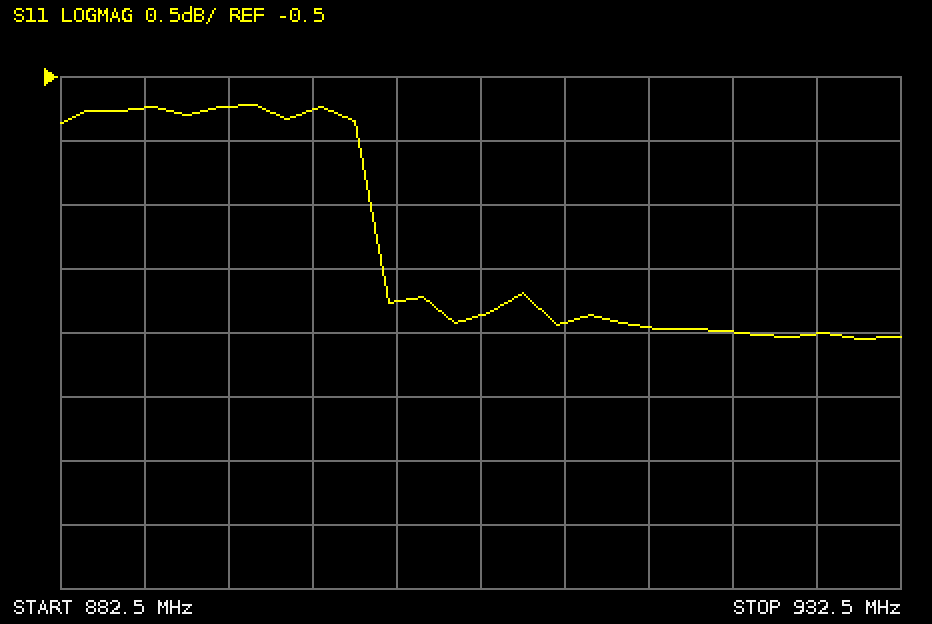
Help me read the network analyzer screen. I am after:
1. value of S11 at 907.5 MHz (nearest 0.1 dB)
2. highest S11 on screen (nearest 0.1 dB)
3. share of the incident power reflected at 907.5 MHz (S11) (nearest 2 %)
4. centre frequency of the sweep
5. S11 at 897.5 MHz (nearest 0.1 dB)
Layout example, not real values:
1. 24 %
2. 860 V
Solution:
1. -2.4 dB
2. -0.7 dB
3. 58 %
4. 907.5 MHz
5. -0.8 dB
